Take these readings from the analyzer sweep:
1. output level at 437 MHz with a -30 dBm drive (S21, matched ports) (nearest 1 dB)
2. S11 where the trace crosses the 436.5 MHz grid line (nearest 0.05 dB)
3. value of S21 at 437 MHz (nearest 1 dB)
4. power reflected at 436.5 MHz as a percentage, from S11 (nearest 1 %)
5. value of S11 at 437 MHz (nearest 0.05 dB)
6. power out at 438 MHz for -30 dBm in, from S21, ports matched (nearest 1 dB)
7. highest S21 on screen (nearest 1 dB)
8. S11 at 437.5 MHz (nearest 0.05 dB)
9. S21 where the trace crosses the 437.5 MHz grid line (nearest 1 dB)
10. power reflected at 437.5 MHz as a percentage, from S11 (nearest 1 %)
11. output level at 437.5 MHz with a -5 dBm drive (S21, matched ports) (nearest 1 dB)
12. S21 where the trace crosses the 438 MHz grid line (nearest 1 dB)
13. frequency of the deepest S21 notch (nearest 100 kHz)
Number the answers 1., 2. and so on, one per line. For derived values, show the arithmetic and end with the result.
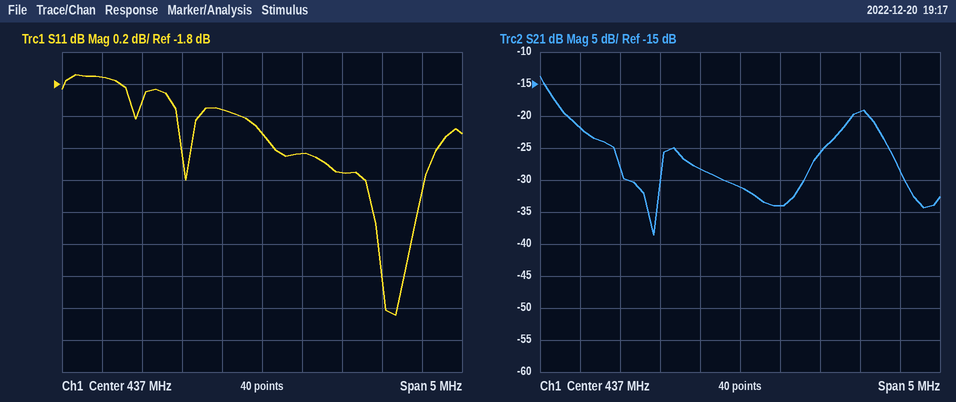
1. -30 dBm + (-31 dB) = -61 dBm
2. -1.95 dB
3. -31 dB
4. 10^(-1.95/10) ≈ 64 %
5. -2.10 dB
6. -30 dBm + (-26 dB) = -56 dBm
7. -14 dB
8. -2.25 dB
9. -34 dB
10. 10^(-2.25/10) ≈ 60 %
11. -5 dBm + (-34 dB) = -39 dBm
12. -26 dB
13. 435.9 MHz
